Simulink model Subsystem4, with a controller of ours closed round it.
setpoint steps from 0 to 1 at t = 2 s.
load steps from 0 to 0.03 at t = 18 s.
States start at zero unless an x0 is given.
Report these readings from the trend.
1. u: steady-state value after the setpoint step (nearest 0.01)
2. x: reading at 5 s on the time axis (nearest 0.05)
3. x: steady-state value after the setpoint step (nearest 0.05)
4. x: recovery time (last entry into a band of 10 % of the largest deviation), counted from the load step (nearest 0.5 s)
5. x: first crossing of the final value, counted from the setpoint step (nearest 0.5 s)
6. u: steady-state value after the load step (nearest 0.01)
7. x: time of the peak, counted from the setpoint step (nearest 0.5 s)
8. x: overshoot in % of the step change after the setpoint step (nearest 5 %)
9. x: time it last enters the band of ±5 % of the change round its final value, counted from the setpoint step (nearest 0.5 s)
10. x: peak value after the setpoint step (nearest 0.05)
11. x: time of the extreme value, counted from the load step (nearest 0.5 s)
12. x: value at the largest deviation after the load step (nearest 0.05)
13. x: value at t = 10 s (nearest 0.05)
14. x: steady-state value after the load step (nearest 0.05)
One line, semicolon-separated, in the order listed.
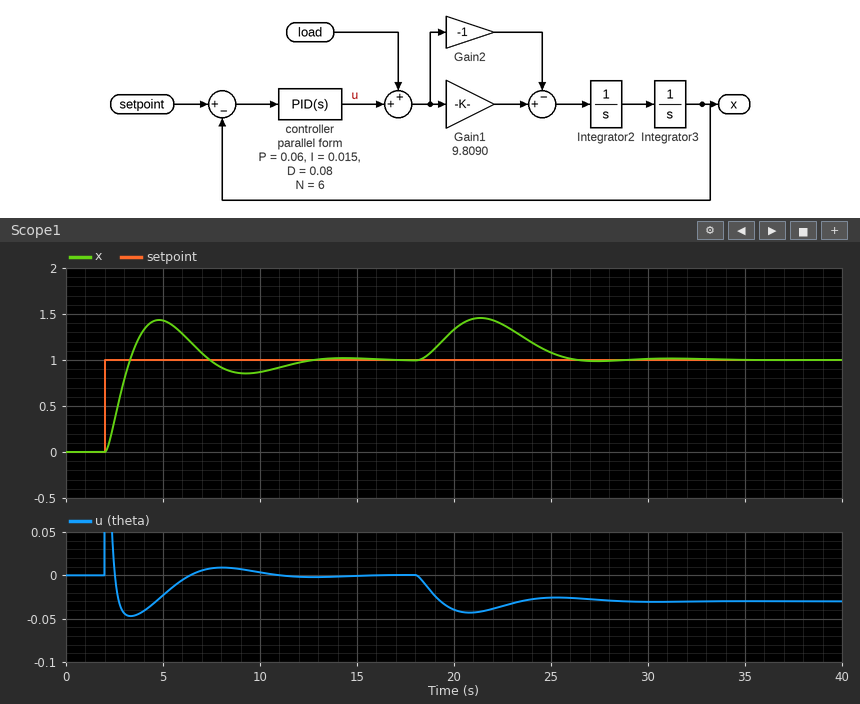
0.00; 1.45; 1.00; 7.5 s; 1.5 s; -0.03; 3.0 s; 45 %; 9.5 s; 1.45; 3.5 s; 1.45; 0.85; 1.00
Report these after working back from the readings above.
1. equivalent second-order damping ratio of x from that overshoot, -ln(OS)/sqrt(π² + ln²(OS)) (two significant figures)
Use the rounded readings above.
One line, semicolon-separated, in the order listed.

0.25
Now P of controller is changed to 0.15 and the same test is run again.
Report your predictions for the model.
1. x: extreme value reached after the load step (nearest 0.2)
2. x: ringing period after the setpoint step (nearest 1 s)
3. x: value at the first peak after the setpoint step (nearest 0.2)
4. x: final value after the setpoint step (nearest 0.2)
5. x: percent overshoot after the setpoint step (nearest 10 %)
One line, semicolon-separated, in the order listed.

1.2; 5 s; 1.6; 1.0; 50 %
